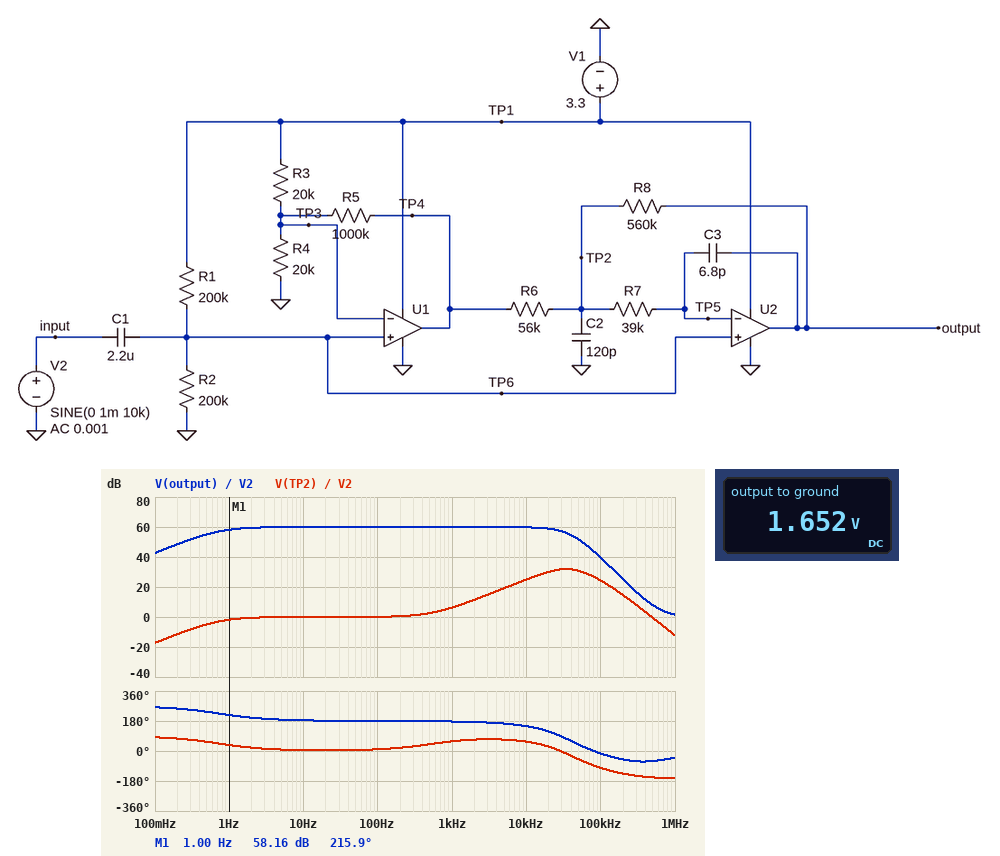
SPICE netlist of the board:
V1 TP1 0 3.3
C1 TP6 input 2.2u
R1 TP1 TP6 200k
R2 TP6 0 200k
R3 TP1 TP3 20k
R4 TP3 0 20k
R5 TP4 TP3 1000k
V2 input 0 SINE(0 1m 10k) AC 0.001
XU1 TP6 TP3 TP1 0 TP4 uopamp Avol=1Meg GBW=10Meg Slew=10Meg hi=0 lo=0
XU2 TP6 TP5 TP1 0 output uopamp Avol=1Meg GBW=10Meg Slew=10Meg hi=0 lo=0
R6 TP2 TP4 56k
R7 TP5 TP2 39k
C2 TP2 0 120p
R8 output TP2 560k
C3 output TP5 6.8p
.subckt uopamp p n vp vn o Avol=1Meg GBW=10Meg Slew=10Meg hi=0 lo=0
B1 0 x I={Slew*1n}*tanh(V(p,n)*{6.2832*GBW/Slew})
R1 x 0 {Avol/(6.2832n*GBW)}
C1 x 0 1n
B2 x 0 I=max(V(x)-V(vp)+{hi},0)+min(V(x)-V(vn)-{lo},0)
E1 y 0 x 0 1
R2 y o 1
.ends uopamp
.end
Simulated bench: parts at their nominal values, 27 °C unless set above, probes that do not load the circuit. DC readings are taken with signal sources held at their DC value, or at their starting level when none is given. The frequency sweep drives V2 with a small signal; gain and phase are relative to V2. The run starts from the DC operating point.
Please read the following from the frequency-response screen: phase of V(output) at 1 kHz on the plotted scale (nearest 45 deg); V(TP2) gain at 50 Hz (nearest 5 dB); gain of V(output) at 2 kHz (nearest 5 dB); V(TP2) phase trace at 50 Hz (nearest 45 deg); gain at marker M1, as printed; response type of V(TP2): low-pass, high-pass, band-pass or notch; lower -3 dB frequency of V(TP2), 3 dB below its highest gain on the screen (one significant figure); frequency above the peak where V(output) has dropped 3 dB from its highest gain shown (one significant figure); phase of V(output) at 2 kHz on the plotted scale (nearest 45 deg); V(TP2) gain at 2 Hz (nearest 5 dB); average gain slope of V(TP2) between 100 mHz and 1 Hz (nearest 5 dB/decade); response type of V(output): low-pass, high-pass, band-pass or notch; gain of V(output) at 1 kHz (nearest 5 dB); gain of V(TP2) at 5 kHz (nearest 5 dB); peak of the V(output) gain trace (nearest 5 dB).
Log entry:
180 deg
0 dB
60 dB
0 deg
58.16 dB
band-pass
20 kHz
30 kHz
180 deg
0 dB
15 dB/decade
band-pass
60 dB
20 dB
60 dB
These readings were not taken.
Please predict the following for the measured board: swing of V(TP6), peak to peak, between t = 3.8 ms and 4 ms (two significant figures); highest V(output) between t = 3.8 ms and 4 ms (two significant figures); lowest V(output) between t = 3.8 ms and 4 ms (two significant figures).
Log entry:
2.0 mV
2.6 V
680 mV
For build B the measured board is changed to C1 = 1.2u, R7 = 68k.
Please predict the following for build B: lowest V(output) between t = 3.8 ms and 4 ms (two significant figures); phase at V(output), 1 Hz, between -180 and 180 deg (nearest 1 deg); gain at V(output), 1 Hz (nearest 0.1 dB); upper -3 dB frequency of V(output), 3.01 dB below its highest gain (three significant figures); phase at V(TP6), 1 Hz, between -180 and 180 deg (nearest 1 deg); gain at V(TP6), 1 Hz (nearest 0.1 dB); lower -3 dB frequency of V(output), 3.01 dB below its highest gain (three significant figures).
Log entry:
700 mV
-127 deg
55.6 dB
23.7 kHz
53 deg
-4.4 dB
1.33 Hz
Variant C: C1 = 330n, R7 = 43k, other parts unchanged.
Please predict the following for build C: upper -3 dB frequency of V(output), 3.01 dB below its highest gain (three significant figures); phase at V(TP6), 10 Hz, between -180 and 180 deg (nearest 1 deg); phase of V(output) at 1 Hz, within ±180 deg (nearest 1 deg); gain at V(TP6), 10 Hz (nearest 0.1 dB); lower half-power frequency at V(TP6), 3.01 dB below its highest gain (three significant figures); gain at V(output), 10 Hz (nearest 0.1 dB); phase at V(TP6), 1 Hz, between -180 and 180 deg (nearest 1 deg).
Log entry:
29.5 kHz
26 deg
-102 deg
-0.9 dB
4.82 Hz
59.1 dB
78 deg
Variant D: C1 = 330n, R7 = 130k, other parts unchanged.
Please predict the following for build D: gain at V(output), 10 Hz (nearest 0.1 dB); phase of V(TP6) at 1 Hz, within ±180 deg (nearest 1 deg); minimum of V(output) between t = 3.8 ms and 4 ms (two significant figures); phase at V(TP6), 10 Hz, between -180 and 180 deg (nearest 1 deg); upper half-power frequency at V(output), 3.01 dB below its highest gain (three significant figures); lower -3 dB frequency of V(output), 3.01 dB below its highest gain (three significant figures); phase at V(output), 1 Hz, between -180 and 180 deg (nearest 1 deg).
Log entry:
59.1 dB
78 deg
790 mV
26 deg
15.5 kHz
4.82 Hz
-102 deg
